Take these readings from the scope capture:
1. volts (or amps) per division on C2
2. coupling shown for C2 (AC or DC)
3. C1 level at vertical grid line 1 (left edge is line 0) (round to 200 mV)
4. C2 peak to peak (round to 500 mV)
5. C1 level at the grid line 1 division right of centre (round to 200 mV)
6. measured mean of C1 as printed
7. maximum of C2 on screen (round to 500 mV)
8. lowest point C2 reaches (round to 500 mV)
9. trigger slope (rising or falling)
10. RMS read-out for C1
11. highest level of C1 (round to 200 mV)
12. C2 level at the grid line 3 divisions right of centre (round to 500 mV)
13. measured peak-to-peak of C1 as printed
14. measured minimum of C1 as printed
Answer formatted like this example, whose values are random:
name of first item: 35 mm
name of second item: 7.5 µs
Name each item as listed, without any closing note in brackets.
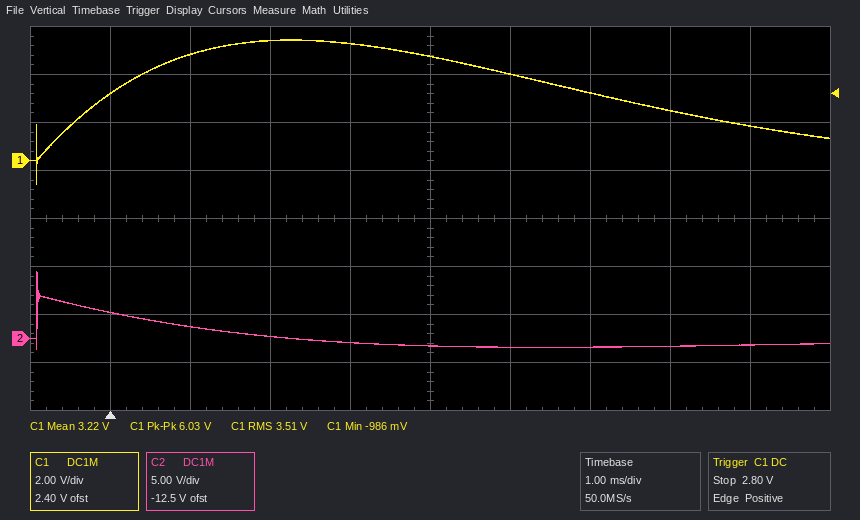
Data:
volts (or amps) per division on C2: 5 V
coupling shown for C2: DC
C1 level at vertical grid line 1 (left edge is line 0): 2.8 V
C2 peak to peak: 8.0 V
C1 level at the grid line 1 division right of centre: 3.6 V
measured mean of C1 as printed: 3.22 V
maximum of C2 on screen: 7.0 V
lowest point C2 reaches: -1.0 V
trigger slope: rising
RMS read-out for C1: 3.51 V
highest level of C1: 5.0 V
C2 level at the grid line 3 divisions right of centre: -1.0 V
measured peak-to-peak of C1 as printed: 6.03 V
measured minimum of C1 as printed: -986 mV
